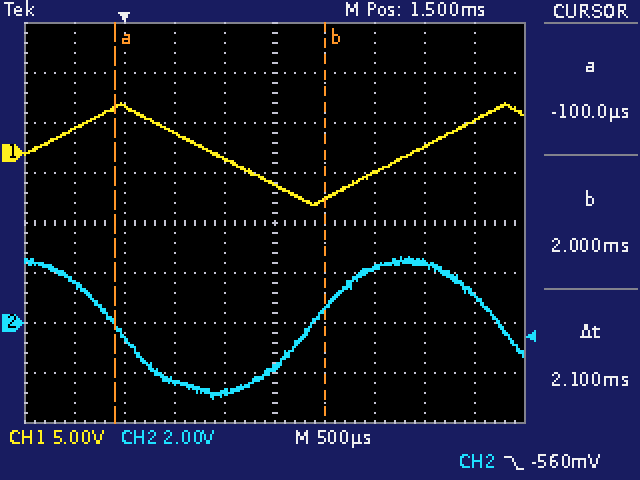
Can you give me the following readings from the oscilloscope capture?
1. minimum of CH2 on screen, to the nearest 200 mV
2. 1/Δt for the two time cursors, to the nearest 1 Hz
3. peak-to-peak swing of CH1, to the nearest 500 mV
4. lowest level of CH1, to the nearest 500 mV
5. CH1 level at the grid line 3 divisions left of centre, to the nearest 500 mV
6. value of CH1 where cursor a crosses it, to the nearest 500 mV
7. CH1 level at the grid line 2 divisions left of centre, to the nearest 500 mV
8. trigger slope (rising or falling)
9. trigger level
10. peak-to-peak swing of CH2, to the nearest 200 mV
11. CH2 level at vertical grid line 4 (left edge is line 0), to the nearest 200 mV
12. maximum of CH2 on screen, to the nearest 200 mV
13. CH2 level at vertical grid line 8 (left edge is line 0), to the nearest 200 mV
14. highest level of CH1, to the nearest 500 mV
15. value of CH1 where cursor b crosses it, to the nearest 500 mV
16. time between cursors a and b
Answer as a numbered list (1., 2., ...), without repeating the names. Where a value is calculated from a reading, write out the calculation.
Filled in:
1. -3.0 V
2. 1 / 2.1 ms ≈ 476 Hz
3. 5.0 V − (-5.0 V) = 10.0 V
4. -5.0 V
5. 4.5 V
6. 4.5 V
7. 2.0 V
8. falling
9. -560 mV
10. 2.6 V − (-3.0 V) = 5.6 V
11. -2.8 V
12. 2.6 V
13. 2.4 V
14. 5.0 V
15. -4.5 V
16. 2.1 ms
